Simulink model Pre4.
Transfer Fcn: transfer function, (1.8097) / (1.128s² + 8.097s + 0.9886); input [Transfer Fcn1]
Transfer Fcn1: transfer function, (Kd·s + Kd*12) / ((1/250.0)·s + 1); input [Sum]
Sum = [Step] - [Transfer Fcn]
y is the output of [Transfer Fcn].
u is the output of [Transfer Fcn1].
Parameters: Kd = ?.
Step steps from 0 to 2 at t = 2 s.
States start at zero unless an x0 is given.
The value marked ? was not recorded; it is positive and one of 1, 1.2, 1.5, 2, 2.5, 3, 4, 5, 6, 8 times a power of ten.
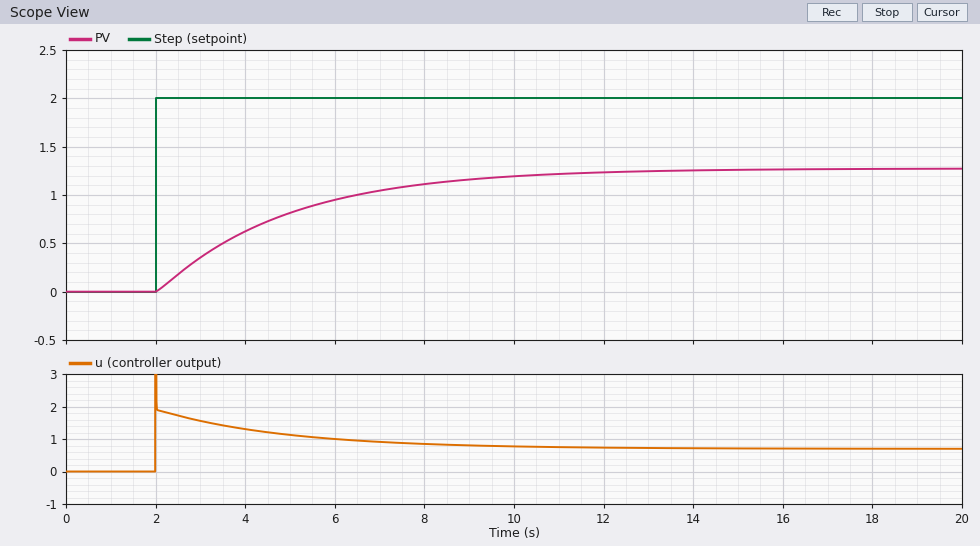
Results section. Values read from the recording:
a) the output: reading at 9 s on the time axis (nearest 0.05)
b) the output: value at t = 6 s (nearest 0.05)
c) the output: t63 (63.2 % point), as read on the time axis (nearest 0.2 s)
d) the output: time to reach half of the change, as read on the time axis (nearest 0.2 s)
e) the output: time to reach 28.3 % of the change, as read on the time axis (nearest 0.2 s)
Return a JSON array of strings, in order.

["1.15", "0.95", "5.0 s", "4.0 s", "3.0 s"]
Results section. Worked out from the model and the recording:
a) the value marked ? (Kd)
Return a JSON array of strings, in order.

["0.08"]
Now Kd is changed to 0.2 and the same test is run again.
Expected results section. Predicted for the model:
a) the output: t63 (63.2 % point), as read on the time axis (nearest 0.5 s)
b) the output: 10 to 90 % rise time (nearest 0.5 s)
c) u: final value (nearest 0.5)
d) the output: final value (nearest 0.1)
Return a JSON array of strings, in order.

["3.5 s", "3.0 s", "1.0", "1.6"]
